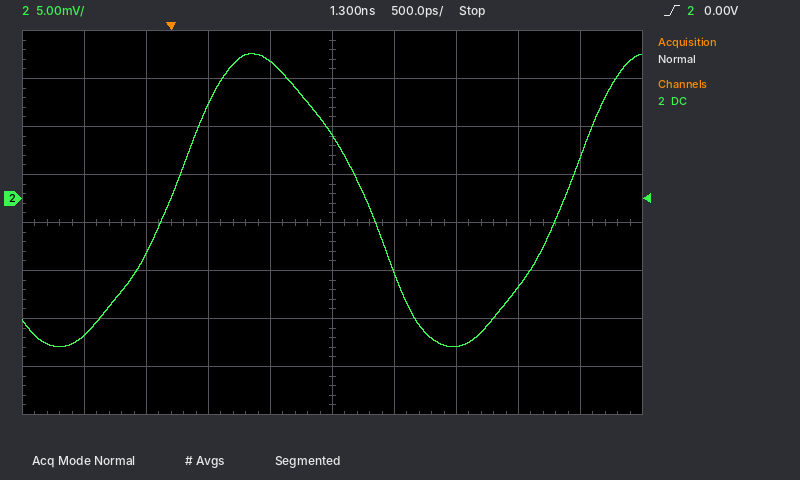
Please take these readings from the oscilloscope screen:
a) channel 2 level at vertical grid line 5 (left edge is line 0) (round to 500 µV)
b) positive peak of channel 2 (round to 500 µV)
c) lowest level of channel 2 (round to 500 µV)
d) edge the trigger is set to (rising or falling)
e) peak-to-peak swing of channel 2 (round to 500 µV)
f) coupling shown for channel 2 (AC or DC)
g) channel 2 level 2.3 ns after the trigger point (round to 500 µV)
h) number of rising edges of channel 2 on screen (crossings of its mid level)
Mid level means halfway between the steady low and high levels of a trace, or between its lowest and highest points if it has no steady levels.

6.5 mV
15.0 mV
-15.5 mV
rising
30.5 mV
DC
-15.5 mV
2
